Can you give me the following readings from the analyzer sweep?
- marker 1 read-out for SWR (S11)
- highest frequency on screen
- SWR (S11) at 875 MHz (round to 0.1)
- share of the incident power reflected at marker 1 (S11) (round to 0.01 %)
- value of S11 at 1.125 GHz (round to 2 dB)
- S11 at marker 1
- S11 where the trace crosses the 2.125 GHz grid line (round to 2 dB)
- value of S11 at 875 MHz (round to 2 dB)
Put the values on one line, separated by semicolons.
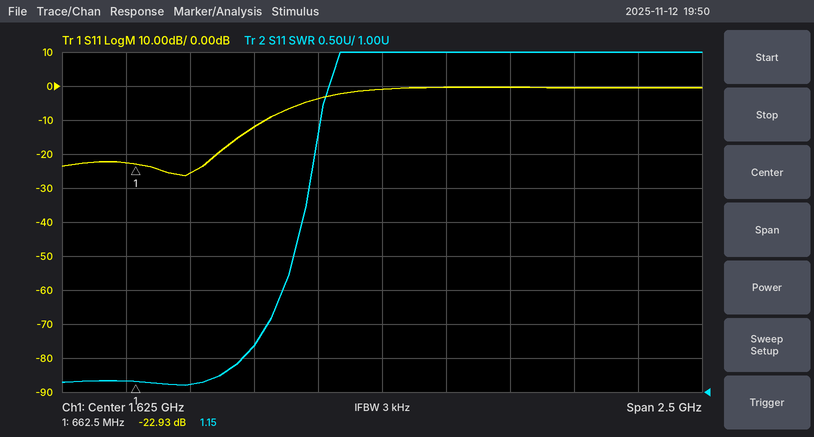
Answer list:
1.15; 2.875 GHz; 1.1; 0.51 %; -12 dB; -22.93 dB; 0 dB; -26 dB
